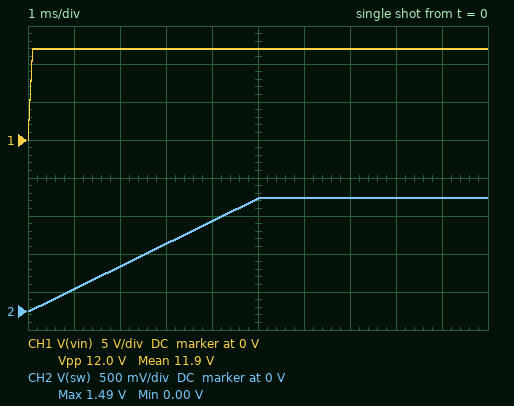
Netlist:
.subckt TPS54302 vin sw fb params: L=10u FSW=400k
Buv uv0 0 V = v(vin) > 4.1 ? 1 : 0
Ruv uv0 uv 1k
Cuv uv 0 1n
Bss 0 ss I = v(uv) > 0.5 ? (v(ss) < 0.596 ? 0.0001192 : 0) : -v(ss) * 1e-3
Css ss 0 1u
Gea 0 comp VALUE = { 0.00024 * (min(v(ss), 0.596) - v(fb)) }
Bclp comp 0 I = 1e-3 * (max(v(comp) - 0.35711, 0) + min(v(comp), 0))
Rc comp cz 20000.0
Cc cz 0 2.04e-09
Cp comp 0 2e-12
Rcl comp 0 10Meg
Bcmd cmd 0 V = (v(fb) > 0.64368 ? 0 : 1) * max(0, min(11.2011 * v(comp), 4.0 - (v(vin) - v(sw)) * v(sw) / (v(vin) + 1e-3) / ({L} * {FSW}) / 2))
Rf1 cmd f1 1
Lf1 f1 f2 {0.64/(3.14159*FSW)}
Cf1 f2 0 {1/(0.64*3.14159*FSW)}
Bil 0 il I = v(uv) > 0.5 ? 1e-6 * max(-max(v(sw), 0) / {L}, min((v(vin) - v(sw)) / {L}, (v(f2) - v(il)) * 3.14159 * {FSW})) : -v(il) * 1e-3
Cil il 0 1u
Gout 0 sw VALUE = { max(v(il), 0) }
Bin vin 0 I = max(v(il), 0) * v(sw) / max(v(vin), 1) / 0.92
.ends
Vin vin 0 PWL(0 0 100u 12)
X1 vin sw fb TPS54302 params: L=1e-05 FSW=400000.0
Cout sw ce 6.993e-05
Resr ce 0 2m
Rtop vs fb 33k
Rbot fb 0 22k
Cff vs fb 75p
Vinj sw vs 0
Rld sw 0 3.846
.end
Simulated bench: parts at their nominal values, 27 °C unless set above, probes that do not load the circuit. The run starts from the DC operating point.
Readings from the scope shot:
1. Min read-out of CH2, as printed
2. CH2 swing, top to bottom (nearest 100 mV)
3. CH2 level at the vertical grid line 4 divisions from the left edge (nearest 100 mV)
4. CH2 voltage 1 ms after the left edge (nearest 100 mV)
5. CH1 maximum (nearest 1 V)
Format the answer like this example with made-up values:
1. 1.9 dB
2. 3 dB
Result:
1. 0.00 V
2. 1.5 V
3. 1.2 V
4. 300 mV
5. 12 V
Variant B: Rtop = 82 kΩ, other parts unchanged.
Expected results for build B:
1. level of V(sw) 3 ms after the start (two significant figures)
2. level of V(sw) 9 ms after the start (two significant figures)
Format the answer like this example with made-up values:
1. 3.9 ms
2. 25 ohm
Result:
1. 1.7 V
2. 2.8 V
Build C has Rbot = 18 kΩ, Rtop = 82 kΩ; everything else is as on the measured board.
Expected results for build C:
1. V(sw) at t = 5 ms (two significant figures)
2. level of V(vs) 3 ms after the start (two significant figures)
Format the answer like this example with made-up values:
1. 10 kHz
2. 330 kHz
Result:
1. 3.3 V
2. 2.0 V
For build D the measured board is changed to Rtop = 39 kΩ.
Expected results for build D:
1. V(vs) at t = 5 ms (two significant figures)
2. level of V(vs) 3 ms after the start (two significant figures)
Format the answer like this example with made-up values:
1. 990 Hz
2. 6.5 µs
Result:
1. 1.6 V
2. 980 mV
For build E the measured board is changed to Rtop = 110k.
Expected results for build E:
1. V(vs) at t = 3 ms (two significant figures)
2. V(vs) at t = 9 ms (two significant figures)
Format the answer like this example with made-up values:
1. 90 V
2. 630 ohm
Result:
1. 2.1 V
2. 3.6 V
